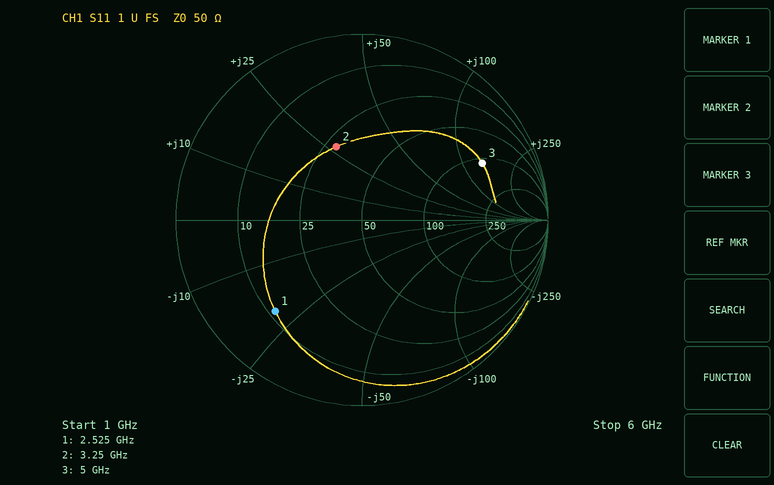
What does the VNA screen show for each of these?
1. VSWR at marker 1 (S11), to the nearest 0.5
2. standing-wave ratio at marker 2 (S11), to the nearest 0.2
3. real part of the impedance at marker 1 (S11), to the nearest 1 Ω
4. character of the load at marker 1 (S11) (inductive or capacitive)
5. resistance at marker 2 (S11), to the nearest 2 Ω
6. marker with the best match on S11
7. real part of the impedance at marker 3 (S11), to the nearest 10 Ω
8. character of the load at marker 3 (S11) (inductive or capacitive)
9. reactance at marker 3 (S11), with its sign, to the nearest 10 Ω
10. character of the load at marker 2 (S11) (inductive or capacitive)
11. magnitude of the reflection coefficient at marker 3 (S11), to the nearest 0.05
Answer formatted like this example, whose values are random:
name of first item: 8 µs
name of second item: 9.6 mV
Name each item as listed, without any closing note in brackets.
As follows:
VSWR at marker 1 (S11), to the nearest 0.5: 5.0
standing-wave ratio at marker 2 (S11), to the nearest 0.2: 2.4
real part of the impedance at marker 1 (S11), to the nearest 1 Ω: 11 Ω
character of the load at marker 1 (S11): capacitive
resistance at marker 2 (S11), to the nearest 2 Ω: 28 Ω
marker with the best match on S11: marker 2
real part of the impedance at marker 3 (S11), to the nearest 10 Ω: 110 Ω
character of the load at marker 3 (S11): inductive
reactance at marker 3 (S11), with its sign, to the nearest 10 Ω: +140 Ω
character of the load at marker 2 (S11): inductive
magnitude of the reflection coefficient at marker 3 (S11), to the nearest 0.05: 0.70
